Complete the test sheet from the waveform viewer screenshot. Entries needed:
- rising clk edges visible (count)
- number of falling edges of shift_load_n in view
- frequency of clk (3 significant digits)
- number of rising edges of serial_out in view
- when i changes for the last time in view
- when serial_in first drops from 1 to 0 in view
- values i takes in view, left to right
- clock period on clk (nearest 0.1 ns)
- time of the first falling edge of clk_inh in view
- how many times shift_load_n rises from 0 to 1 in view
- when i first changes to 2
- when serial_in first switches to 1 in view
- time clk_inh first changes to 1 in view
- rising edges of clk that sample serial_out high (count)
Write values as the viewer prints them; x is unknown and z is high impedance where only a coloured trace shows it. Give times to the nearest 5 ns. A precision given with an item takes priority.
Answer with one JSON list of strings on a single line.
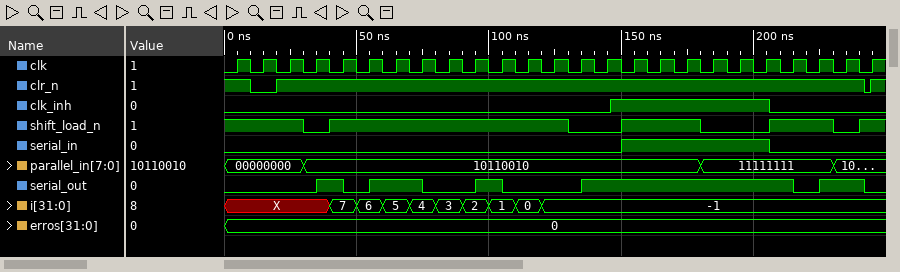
["25", "4", "100 MHz", "5", "120 ns", "205 ns", "X, 7, 6, 5, 4, 3, 2, 1, 0, -1", "10 ns", "205 ns", "4", "90 ns", "150 ns", "145 ns", "13"]
